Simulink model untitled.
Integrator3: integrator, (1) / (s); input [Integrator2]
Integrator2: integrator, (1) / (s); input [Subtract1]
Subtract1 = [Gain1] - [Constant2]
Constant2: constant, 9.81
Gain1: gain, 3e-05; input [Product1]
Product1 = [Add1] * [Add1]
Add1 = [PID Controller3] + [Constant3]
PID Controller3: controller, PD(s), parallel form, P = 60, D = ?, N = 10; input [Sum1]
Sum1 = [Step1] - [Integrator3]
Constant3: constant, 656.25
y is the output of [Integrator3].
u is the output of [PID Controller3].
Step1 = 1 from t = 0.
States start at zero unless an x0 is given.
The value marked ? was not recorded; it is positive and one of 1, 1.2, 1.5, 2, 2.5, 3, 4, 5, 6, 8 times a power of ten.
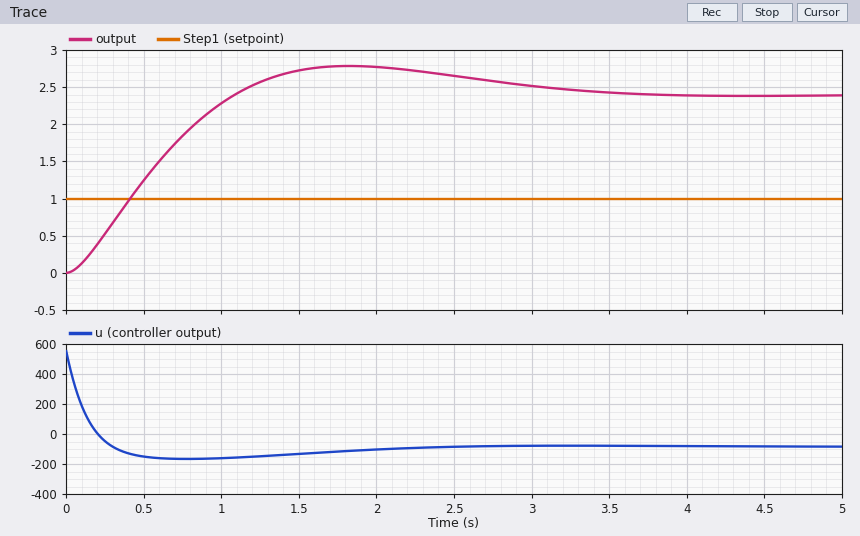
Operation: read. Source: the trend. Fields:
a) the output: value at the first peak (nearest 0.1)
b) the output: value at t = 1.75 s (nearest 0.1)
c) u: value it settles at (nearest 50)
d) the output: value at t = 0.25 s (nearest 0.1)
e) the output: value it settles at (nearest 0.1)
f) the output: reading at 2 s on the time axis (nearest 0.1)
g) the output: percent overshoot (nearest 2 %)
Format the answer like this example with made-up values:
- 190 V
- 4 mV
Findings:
- 2.8
- 2.8
- -100
- 0.5
- 2.4
- 2.8
- 16 %
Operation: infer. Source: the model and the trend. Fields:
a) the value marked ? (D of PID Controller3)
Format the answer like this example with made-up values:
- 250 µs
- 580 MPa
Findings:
- 50
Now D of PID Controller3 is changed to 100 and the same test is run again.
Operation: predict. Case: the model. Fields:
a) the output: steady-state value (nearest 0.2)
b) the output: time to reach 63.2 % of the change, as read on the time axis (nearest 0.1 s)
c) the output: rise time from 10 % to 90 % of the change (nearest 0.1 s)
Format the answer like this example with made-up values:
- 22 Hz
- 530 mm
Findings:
- 2.4
- 0.4 s
- 0.7 s
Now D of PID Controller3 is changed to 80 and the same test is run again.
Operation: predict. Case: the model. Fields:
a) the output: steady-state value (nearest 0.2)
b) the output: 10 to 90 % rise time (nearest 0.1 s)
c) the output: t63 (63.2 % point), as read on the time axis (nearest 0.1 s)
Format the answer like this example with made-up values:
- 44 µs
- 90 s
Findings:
- 2.4
- 0.8 s
- 0.5 s
